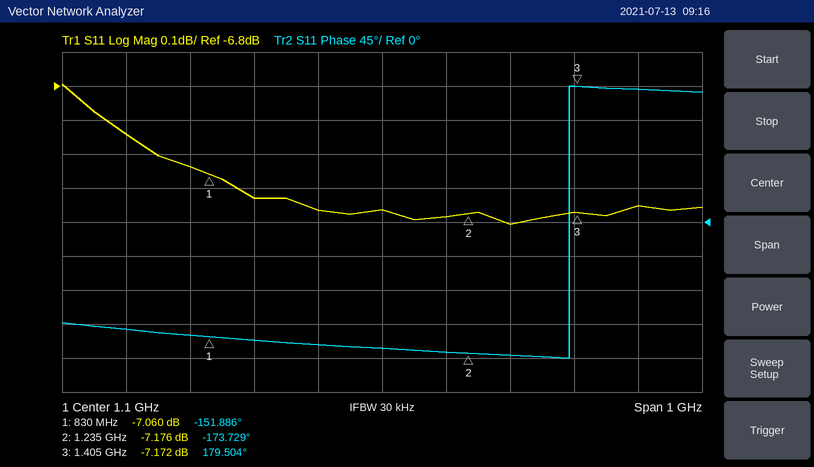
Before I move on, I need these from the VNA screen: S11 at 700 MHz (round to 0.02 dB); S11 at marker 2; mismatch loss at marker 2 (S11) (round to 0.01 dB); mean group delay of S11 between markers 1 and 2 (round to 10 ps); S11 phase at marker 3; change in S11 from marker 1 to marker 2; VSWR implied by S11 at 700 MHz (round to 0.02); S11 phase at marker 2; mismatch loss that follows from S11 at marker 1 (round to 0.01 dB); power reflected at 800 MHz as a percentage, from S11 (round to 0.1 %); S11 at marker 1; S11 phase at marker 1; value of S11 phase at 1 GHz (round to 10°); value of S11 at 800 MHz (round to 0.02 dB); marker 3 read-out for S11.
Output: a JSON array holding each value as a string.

["-6.94 dB", "-7.176 dB", "0.92 dB", "150 ps", "179.504°", "-0.116 dB", "2.64", "-173.729°", "0.95 dB", "19.8 %", "-7.060 dB", "-151.886°", "-160°", "-7.04 dB", "-7.172 dB"]
